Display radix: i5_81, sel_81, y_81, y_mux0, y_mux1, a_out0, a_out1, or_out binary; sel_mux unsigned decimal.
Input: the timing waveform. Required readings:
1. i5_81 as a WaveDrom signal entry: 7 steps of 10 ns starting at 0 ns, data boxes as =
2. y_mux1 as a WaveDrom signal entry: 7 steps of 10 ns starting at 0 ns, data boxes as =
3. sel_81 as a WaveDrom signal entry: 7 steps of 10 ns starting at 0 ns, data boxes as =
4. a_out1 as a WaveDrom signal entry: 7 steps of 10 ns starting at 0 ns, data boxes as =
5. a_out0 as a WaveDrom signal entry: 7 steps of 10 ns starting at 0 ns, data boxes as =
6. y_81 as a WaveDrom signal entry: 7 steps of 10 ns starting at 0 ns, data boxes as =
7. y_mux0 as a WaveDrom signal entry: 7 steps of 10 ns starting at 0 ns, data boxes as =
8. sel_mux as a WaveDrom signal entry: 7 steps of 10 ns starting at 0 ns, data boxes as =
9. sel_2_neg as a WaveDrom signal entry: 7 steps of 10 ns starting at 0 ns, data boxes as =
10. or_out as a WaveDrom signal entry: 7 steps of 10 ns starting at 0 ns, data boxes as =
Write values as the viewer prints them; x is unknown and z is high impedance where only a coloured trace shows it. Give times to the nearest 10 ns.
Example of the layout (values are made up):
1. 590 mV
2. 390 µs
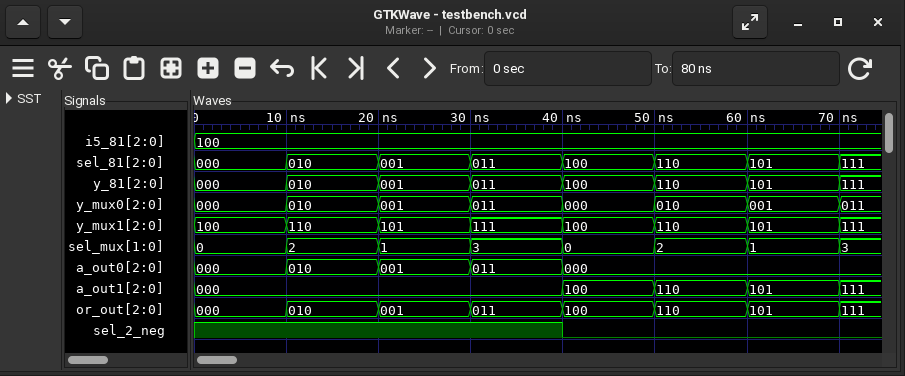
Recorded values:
1. {name: 'i5_81', wave: '=......', data: '100'}
2. {name: 'y_mux1', wave: '=======', data: '100 110 101 111 100 110 101'}
3. {name: 'sel_81', wave: '=======', data: '000 010 001 011 100 110 101'}
4. {name: 'a_out1', wave: '=...===', data: '000 100 110 101'}
5. {name: 'a_out0', wave: '=====..', data: '000 010 001 011 000'}
6. {name: 'y_81', wave: '=======', data: '000 010 001 011 100 110 101'}
7. {name: 'y_mux0', wave: '=======', data: '000 010 001 011 000 010 001'}
8. {name: 'sel_mux', wave: '=======', data: '0 2 1 3 0 2 1'}
9. {name: 'sel_2_neg', wave: '1...0..'}
10. {name: 'or_out', wave: '=======', data: '000 010 001 011 100 110 101'}
